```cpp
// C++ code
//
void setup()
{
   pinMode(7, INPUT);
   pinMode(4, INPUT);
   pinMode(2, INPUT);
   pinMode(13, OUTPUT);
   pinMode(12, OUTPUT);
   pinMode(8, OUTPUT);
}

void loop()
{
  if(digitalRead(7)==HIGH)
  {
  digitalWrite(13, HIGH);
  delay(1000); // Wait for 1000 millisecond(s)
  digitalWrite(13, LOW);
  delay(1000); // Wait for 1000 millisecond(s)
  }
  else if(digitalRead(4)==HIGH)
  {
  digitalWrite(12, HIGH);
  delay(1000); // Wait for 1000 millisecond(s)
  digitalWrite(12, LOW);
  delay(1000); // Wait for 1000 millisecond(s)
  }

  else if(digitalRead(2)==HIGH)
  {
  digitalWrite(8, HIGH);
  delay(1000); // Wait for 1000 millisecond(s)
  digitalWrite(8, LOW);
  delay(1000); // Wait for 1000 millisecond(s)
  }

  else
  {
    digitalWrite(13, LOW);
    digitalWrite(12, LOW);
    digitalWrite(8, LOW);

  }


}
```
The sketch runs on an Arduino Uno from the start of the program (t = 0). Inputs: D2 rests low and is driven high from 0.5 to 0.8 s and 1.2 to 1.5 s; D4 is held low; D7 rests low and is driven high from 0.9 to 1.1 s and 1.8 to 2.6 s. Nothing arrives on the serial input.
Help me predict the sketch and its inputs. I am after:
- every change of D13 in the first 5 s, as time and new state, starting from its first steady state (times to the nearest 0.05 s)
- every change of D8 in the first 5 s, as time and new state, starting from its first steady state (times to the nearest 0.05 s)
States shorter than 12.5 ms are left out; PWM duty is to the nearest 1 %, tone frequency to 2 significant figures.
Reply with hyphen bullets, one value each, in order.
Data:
- 0 s low; 2.5 s high; 3.5 s low
- 0 s low; 0.5 s high; 1.5 s low
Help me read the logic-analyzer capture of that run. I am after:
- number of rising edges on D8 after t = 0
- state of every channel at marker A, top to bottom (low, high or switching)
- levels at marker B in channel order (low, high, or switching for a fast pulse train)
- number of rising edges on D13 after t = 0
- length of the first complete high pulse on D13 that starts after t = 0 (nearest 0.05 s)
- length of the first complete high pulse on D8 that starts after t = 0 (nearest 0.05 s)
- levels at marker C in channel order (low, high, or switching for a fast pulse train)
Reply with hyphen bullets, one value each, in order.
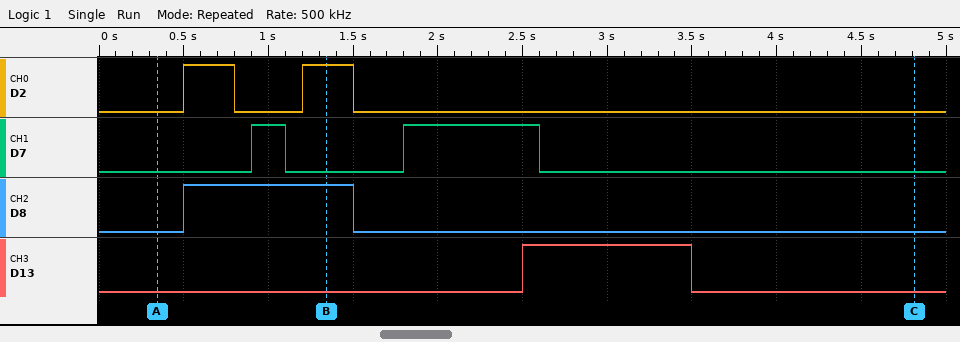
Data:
- 1
- D2 low, D7 low, D8 low, D13 low
- D2 high, D7 low, D8 high, D13 low
- 1
- 1.00 s
- 1.00 s
- D2 low, D7 low, D8 low, D13 low
